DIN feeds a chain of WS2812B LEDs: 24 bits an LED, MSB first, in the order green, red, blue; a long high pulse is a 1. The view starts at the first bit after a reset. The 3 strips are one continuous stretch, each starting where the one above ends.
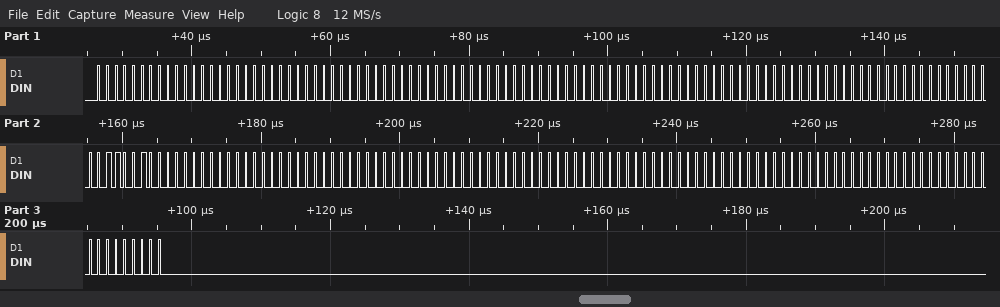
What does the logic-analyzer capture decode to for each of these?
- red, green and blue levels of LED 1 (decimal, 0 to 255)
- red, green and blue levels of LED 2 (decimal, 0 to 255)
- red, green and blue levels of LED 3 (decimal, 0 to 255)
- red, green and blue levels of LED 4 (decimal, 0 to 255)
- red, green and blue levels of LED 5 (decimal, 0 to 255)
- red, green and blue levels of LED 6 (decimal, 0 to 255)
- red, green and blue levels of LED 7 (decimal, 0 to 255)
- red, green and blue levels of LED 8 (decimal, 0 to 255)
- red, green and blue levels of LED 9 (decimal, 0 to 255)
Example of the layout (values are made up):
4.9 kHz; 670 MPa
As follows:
0, 0, 0; 0, 0, 0; 0, 0, 0; 0, 0, 0; 100, 0, 0; 0, 0, 0; 0, 0, 0; 0, 0, 0; 0, 0, 0
